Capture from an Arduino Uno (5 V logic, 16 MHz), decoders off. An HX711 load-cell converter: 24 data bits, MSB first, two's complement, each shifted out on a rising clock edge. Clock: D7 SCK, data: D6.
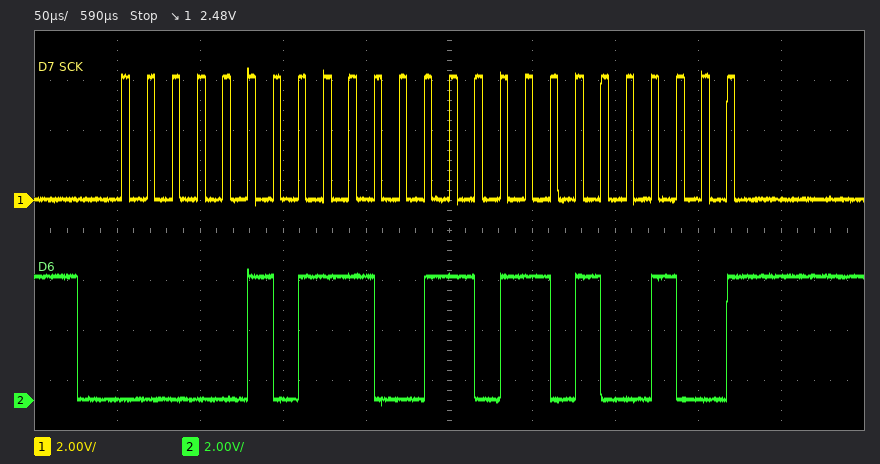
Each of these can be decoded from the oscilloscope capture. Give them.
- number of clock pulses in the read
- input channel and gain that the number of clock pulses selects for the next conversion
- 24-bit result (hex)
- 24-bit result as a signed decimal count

25
channel A, gain 128
0x05CDA4
380324
